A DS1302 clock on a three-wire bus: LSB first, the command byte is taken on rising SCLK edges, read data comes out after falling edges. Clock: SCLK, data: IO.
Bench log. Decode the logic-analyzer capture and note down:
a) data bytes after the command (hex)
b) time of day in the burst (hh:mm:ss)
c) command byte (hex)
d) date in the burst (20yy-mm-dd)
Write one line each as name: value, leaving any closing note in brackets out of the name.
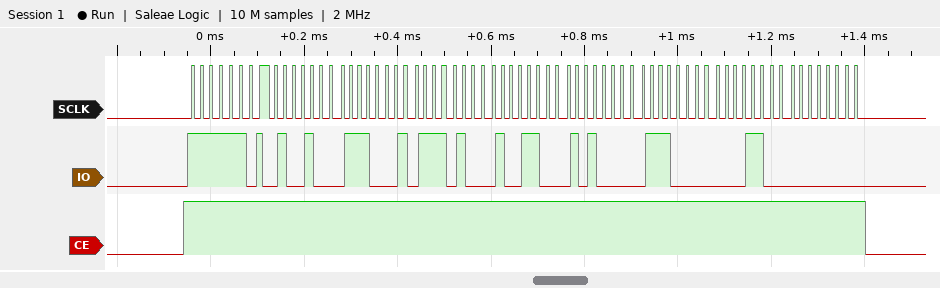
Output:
data bytes after the command: 12 47 17 19 05 07 18 00
time of day in the burst: 17:47:12
command byte: 0xBF
date in the burst: 2018-05-19
